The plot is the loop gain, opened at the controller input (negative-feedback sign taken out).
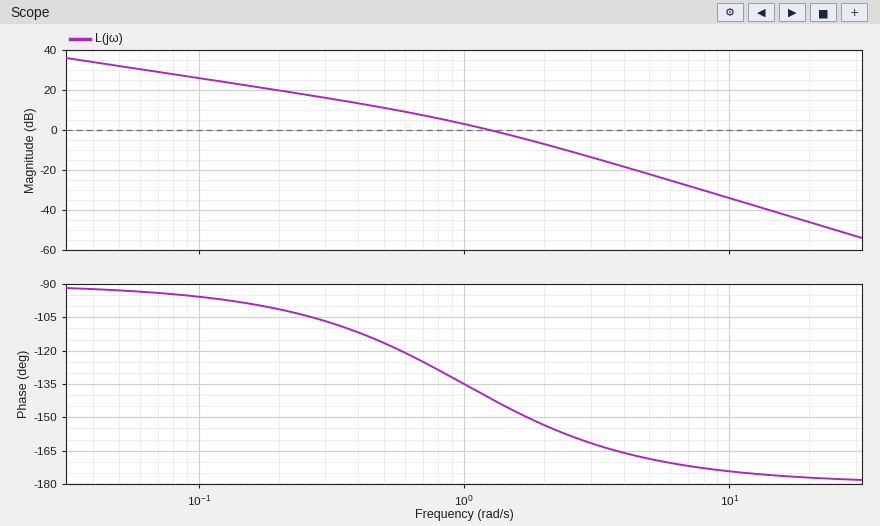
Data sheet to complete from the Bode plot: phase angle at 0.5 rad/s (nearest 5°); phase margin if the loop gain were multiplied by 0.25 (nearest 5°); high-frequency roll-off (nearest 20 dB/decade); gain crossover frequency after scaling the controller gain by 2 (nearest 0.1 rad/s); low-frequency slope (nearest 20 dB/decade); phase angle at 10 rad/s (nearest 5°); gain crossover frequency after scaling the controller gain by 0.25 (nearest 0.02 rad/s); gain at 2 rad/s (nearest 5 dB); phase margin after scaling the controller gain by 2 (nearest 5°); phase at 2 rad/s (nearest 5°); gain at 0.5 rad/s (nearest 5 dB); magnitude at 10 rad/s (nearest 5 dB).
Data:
-115°
65°
-40 dB/decade
1.9 rad/s
-20 dB/decade
-175°
0.46 rad/s
-5 dB
30°
-155°
10 dB
-35 dB
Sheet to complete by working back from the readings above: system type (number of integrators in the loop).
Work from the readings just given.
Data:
1
